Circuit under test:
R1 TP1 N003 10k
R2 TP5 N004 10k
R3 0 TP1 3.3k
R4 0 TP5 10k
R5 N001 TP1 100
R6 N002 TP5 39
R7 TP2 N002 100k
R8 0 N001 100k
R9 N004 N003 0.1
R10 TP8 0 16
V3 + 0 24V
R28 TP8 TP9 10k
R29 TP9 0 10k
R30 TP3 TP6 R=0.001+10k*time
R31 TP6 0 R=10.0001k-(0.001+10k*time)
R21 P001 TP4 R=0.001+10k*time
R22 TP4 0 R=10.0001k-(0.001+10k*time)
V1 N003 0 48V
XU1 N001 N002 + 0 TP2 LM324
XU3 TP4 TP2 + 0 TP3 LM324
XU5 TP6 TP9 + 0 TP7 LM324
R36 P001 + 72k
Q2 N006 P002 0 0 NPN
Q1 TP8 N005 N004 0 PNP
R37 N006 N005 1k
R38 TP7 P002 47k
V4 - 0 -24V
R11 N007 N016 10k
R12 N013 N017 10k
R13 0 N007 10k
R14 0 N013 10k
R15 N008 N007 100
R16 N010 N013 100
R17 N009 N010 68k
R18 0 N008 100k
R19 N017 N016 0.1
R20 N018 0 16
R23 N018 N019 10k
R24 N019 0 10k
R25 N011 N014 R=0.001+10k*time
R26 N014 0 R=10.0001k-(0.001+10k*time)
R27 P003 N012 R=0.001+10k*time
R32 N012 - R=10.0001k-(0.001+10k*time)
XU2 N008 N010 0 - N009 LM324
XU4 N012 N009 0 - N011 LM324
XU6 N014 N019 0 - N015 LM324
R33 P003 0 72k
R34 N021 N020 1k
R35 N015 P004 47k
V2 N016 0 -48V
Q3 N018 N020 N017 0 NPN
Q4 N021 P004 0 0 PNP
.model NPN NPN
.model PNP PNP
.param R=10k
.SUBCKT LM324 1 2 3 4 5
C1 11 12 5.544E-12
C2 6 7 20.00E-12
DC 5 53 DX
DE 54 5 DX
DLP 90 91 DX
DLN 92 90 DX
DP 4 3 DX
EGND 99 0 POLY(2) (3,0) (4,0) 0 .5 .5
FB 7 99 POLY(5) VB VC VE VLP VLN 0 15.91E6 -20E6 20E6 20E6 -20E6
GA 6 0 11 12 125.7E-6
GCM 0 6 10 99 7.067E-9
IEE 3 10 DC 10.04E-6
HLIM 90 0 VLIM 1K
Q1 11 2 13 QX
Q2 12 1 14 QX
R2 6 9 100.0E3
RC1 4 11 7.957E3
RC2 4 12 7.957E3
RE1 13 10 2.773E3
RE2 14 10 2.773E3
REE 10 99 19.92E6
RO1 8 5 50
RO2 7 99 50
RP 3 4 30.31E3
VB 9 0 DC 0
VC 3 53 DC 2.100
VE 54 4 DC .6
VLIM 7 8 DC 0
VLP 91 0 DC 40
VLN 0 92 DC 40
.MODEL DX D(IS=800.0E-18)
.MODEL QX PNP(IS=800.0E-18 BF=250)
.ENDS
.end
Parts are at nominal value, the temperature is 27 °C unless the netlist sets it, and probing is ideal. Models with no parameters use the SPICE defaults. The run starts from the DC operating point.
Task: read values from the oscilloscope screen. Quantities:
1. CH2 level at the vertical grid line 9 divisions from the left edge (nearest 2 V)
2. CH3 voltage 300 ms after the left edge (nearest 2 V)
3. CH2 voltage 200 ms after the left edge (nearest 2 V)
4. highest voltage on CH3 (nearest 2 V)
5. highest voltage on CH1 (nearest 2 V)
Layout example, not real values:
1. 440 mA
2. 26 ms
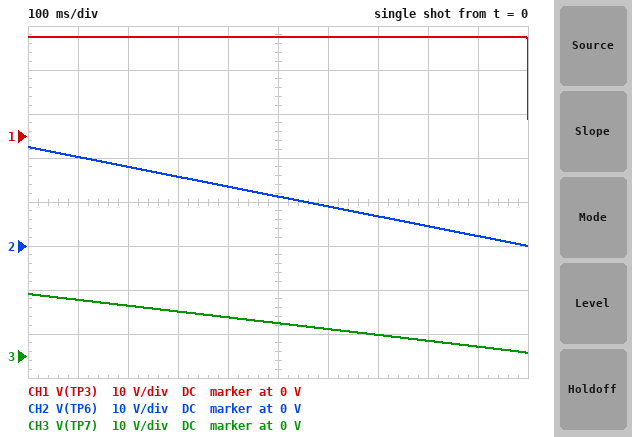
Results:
1. 2 V
2. 10 V
3. 18 V
4. 14 V
5. 22 V
